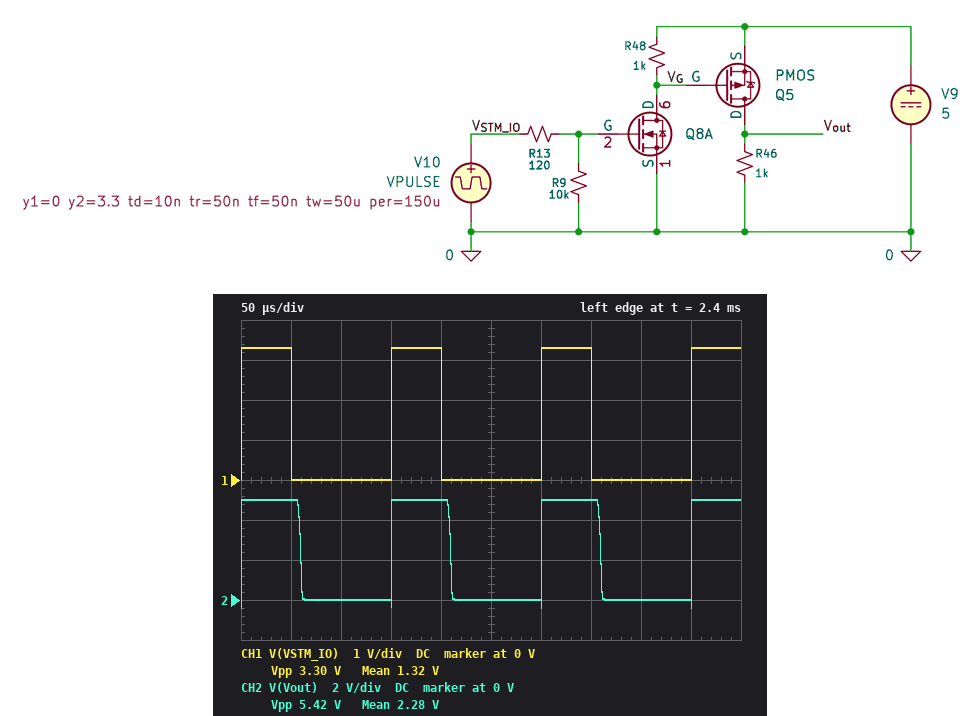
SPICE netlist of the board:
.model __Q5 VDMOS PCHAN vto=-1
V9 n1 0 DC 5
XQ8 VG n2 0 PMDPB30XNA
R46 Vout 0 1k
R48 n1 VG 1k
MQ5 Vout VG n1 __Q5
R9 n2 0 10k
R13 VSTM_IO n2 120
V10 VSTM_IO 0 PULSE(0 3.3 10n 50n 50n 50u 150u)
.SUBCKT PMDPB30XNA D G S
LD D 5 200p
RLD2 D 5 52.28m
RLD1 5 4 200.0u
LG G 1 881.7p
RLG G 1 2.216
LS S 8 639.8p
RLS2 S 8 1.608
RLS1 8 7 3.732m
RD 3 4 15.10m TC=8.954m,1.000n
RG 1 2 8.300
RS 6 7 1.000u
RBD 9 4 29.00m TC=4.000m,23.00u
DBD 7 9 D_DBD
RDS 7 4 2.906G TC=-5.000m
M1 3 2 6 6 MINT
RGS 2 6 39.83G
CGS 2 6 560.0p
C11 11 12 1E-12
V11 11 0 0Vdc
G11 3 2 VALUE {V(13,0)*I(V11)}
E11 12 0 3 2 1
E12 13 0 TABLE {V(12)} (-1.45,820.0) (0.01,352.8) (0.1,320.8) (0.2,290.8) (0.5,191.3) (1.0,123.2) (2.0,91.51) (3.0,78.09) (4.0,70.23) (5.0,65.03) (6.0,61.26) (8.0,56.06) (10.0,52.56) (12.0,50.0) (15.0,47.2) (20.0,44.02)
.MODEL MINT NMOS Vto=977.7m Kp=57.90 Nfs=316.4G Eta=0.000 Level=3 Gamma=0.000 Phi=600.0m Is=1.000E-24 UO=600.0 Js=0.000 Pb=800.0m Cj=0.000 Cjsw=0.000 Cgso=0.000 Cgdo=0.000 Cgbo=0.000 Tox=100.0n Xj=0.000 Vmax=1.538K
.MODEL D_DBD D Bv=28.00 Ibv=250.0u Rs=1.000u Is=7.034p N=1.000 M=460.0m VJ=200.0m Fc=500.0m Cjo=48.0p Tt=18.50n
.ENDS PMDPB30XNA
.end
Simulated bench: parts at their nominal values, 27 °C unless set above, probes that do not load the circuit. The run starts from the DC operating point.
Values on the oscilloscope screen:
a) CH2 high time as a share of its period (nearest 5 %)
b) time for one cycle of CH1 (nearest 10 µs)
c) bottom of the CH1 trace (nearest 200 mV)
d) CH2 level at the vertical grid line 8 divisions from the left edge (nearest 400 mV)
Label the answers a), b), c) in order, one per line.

a) 40 %
b) 150 µs
c) 0 V
d) 0 V
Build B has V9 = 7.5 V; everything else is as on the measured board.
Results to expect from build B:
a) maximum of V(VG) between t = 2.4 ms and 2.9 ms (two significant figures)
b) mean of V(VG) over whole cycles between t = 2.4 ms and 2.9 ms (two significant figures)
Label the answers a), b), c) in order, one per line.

a) 7.5 V
b) 4.8 V
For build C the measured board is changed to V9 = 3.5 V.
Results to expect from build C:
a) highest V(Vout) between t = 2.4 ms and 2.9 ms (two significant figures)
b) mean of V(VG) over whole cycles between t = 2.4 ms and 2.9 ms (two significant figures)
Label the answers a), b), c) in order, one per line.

a) 3.5 V
b) 2.2 V
